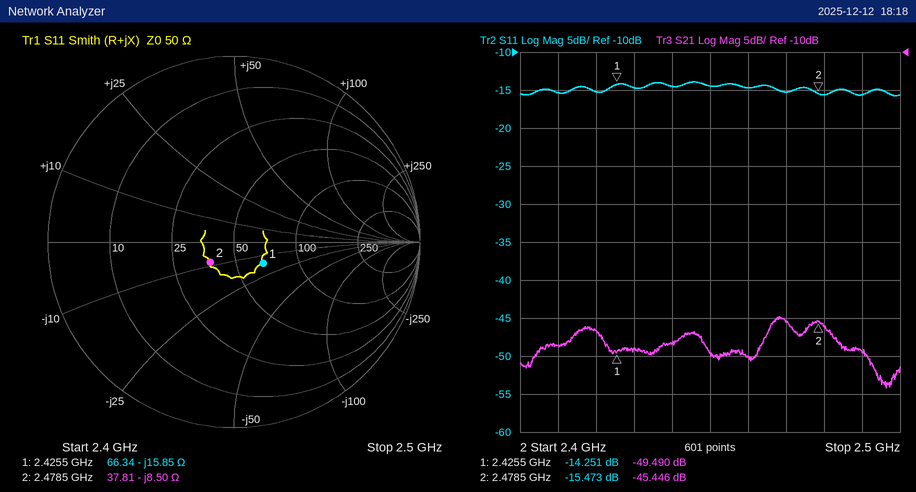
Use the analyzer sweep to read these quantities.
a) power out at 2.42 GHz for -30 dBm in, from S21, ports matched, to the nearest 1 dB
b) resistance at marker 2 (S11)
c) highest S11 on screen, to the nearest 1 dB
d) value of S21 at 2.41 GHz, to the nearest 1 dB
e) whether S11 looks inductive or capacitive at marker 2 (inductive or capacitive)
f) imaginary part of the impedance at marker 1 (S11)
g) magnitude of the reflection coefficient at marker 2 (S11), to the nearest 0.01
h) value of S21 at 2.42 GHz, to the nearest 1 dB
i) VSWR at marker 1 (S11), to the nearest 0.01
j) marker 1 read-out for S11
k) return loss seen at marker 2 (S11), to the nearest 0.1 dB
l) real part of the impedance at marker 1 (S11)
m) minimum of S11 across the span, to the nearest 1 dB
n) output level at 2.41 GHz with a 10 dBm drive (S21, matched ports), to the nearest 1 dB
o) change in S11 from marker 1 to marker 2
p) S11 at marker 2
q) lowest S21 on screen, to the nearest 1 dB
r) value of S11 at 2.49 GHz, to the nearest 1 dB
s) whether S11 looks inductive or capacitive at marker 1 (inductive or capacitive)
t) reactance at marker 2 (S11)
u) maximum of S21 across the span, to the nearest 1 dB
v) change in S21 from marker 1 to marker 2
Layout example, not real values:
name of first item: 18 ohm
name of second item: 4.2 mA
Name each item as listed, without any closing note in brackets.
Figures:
power out at 2.42 GHz for -30 dBm in, from S21, ports matched, to the nearest 1 dB: -77 dBm
resistance at marker 2: 37.81 Ω
highest S11 on screen, to the nearest 1 dB: -14 dB
value of S21 at 2.41 GHz, to the nearest 1 dB: -49 dB
whether S11 looks inductive or capacitive at marker 2: capacitive
imaginary part of the impedance at marker 1: -15.85 Ω
magnitude of the reflection coefficient at marker 2 (S11), to the nearest 0.01: 0.17
value of S21 at 2.42 GHz, to the nearest 1 dB: -47 dB
VSWR at marker 1 (S11), to the nearest 0.01: 1.48
marker 1 read-out for S11: -14.251 dB
return loss seen at marker 2 (S11), to the nearest 0.1 dB: 15.5 dB
real part of the impedance at marker 1: 66.34 Ω
minimum of S11 across the span, to the nearest 1 dB: -16 dB
output level at 2.41 GHz with a 10 dBm drive (S21, matched ports), to the nearest 1 dB: -39 dBm
change in S11 from marker 1 to marker 2: -1.222 dB
S11 at marker 2: -15.473 dB
lowest S21 on screen, to the nearest 1 dB: -54 dB
value of S11 at 2.49 GHz, to the nearest 1 dB: -16 dB
whether S11 looks inductive or capacitive at marker 1: capacitive
reactance at marker 2: -8.50 Ω
maximum of S21 across the span, to the nearest 1 dB: -45 dB
change in S21 from marker 1 to marker 2: 4.044 dB
